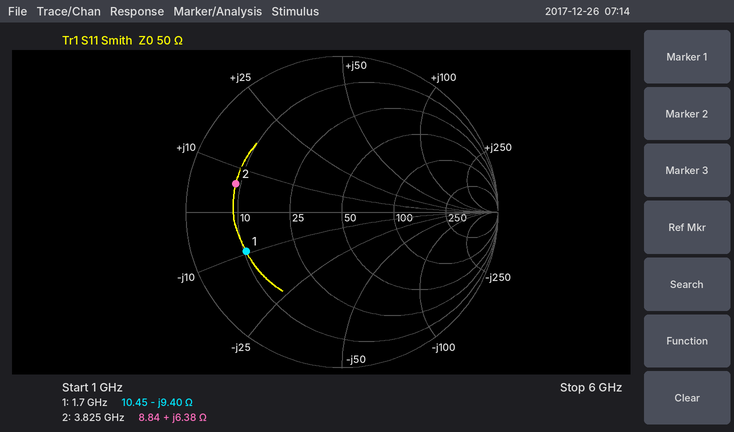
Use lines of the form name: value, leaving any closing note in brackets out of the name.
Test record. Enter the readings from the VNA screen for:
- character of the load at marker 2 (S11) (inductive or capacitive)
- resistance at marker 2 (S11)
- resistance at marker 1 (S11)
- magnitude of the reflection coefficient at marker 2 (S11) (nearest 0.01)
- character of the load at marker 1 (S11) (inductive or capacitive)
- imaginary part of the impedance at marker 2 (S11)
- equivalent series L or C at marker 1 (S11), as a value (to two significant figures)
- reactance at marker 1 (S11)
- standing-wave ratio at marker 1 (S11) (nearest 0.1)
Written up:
character of the load at marker 2 (S11): inductive
resistance at marker 2: 8.84 Ω
resistance at marker 1: 10.45 Ω
magnitude of the reflection coefficient at marker 2 (S11): 0.70
character of the load at marker 1 (S11): capacitive
imaginary part of the impedance at marker 2: +6.38 Ω
equivalent series L or C at marker 1 (S11), as a value: 10.0 pF
reactance at marker 1: -9.40 Ω
standing-wave ratio at marker 1 (S11): 5.0
